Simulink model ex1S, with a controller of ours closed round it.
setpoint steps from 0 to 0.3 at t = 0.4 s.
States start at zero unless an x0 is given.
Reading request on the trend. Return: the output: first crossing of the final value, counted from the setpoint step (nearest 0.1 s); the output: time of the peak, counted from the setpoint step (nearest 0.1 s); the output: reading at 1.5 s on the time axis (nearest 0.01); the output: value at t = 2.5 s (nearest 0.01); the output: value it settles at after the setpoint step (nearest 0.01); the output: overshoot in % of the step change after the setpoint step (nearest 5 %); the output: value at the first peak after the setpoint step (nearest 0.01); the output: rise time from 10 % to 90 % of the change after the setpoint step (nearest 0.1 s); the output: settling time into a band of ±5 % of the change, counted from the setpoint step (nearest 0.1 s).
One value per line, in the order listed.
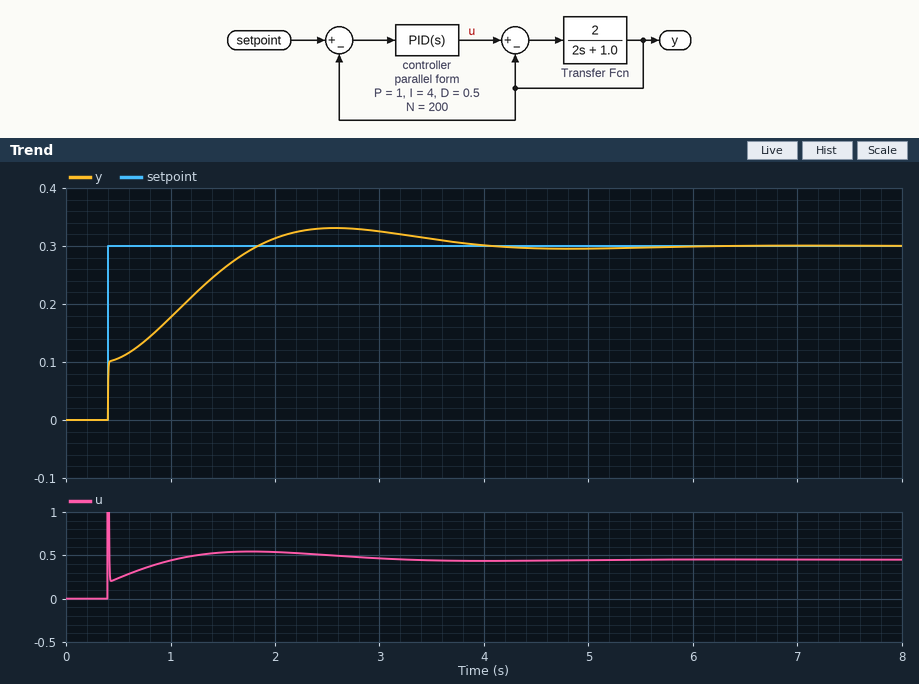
1.4 s
2.2 s
0.26
0.33
0.30
10 %
0.33
1.2 s
3.0 s
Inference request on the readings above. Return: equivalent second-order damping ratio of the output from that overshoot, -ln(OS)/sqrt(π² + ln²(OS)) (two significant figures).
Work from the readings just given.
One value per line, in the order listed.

0.59
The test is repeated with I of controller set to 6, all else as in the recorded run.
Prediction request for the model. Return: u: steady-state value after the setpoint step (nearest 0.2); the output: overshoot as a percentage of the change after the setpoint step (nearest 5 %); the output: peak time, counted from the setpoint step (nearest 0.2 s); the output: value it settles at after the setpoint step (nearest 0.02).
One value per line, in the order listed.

0.4
15 %
1.6 s
0.30
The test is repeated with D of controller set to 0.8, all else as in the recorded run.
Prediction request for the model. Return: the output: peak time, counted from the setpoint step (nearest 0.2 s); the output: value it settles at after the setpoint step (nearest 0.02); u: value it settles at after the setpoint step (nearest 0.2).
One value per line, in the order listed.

2.4 s
0.30
0.4
